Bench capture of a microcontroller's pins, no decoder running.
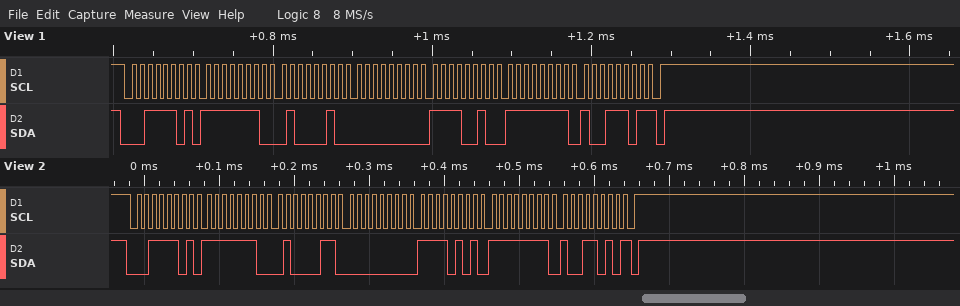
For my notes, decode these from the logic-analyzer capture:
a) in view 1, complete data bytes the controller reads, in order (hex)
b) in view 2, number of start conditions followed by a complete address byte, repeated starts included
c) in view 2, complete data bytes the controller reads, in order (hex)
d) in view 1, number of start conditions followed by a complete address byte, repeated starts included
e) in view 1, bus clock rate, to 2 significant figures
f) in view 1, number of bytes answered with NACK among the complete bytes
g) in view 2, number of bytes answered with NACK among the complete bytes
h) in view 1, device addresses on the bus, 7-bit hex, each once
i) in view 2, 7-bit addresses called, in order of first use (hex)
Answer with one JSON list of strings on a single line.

["FE 42 00 F2 FF 9D", "1", "FE 43 00 F5 FF 9A", "1", "100 kHz", "1", "1", "0x1E", "0x1E"]
